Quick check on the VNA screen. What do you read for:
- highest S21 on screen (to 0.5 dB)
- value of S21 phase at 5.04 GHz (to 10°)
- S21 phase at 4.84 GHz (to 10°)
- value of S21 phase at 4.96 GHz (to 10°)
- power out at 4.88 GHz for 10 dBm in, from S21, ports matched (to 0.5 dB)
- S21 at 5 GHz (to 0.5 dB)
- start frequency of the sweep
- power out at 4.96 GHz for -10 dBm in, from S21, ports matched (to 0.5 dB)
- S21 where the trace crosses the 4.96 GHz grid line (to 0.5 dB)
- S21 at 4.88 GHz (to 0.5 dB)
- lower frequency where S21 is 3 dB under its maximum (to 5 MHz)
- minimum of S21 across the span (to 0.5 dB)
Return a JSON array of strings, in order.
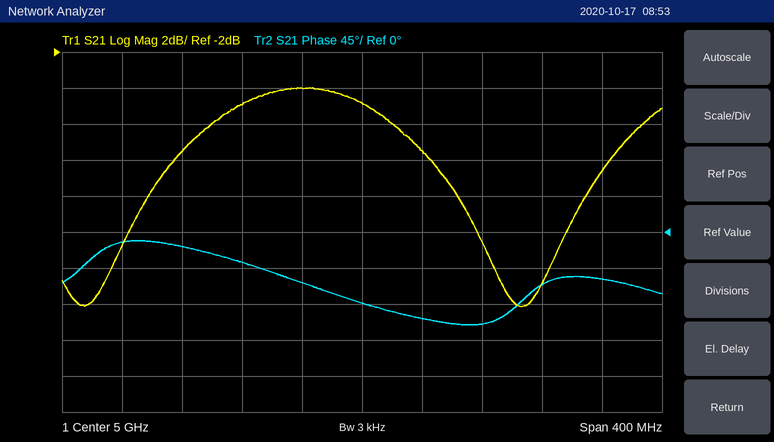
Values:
["-4.0 dB", "-110°", "-10°", "-60°", "2.5 dBm", "-5.0 dB", "4.8 GHz", "-14.0 dBm", "-4.0 dB", "-7.5 dB", "4.885 GHz", "-16.0 dB"]
